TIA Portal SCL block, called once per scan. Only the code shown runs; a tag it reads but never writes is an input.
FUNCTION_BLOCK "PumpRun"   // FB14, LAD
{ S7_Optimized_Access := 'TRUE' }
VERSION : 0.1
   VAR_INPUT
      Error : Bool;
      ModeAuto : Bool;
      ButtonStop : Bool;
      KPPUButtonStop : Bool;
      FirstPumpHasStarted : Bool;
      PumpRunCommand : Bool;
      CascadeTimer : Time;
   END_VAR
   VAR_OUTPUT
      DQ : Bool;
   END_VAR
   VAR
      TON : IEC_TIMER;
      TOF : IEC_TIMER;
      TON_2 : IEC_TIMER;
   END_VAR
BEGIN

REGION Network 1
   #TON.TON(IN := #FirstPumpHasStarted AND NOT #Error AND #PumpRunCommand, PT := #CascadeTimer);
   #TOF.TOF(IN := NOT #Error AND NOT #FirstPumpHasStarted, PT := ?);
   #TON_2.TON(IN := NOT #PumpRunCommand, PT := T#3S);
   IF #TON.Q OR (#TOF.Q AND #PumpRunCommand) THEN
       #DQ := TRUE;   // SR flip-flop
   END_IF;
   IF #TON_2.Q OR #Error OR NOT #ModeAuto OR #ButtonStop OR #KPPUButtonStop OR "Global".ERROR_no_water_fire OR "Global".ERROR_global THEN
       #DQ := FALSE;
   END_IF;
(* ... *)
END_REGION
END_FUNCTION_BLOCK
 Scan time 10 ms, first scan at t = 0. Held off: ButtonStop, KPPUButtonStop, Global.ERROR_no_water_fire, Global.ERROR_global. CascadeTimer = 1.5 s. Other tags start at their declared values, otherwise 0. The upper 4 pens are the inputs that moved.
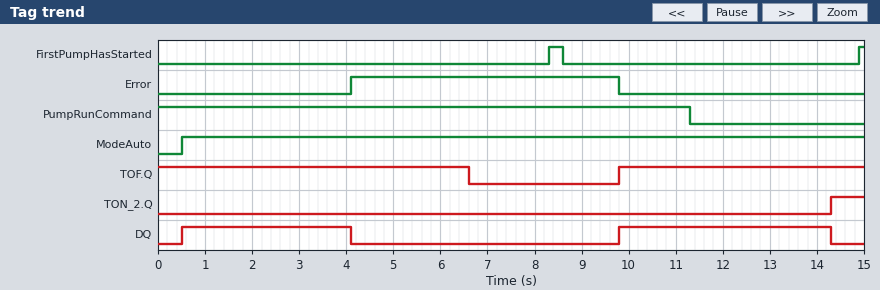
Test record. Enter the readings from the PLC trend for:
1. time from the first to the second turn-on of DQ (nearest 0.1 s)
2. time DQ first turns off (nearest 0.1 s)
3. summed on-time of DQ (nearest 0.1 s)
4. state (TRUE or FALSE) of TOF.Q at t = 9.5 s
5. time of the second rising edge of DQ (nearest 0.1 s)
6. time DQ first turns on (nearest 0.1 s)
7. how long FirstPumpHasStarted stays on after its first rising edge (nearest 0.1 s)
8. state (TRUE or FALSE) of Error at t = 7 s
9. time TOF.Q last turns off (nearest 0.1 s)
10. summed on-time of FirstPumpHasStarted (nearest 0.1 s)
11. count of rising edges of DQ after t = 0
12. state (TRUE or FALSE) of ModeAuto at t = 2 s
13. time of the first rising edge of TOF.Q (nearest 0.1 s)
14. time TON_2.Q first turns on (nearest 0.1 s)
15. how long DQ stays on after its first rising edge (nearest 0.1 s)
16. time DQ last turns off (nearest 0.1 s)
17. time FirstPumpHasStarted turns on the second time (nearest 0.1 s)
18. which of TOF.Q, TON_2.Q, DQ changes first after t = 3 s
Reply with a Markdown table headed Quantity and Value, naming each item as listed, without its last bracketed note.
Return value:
| Quantity | Value |
|---|---|
| time from the first to the second turn-on of DQ | 9.3 s |
| time DQ first turns off | 4.1 s |
| summed on-time of DQ | 8.1 s |
| state (TRUE or FALSE) of TOF.Q at t = 9.5 s | FALSE |
| time of the second rising edge of DQ | 9.8 s |
| time DQ first turns on | 0.5 s |
| how long FirstPumpHasStarted stays on after its first rising edge | 0.3 s |
| state (TRUE or FALSE) of Error at t = 7 s | TRUE |
| time TOF.Q last turns off | 6.6 s |
| summed on-time of FirstPumpHasStarted | 0.4 s |
| count of rising edges of DQ after t = 0 | 2 |
| state (TRUE or FALSE) of ModeAuto at t = 2 s | TRUE |
| time of the first rising edge of TOF.Q | 9.8 s |
| time TON_2.Q first turns on | 14.3 s |
| how long DQ stays on after its first rising edge | 3.6 s |
| time DQ last turns off | 14.3 s |
| time FirstPumpHasStarted turns on the second time | 14.9 s |
| which of TOF.Q, TON_2.Q, DQ changes first after t = 3 s | DQ |
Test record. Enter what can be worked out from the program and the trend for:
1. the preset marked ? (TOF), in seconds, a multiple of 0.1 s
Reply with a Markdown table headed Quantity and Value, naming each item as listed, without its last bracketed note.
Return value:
| Quantity | Value |
|---|---|
| the preset marked ? (TOF), in seconds, a multiple of 0.1 s | 2.5 s |
